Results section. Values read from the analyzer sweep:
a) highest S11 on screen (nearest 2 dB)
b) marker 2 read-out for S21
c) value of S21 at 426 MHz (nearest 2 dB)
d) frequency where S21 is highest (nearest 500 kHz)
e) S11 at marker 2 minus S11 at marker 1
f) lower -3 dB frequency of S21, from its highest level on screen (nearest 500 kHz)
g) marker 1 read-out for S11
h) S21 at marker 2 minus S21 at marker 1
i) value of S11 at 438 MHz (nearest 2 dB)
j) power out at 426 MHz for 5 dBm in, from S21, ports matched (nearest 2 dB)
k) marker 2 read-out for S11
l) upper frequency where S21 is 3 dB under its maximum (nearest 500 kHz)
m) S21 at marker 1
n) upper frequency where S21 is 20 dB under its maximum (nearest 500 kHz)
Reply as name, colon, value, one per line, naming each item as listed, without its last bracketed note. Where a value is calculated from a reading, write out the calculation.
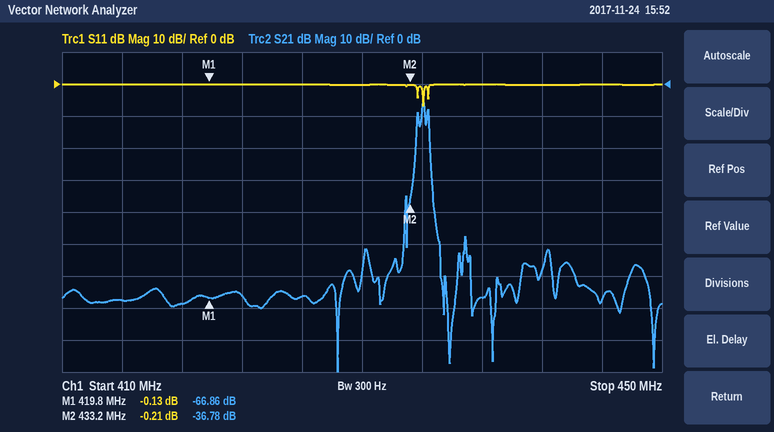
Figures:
highest S11 on screen: 0 dB
marker 2 read-out for S21: -36.78 dB
value of S21 at 426 MHz: -66 dB
frequency where S21 is highest: 434.0 MHz
S11 at marker 2 minus S11 at marker 1: -0.21 − (-0.13) = -0.08 dB
lower -3 dB frequency of S21, from its highest level on screen: 434.0 MHz
marker 1 read-out for S11: -0.13 dB
S21 at marker 2 minus S21 at marker 1: -36.78 − (-66.86) = 30.08 dB
value of S11 at 438 MHz: 0 dB
power out at 426 MHz for 5 dBm in, from S21, ports matched: 5 dBm + (-66 dB) = -62 dBm
marker 2 read-out for S11: -0.21 dB
upper frequency where S21 is 3 dB under its maximum: 434.0 MHz
S21 at marker 1: -66.86 dB
upper frequency where S21 is 20 dB under its maximum: 434.5 MHz
